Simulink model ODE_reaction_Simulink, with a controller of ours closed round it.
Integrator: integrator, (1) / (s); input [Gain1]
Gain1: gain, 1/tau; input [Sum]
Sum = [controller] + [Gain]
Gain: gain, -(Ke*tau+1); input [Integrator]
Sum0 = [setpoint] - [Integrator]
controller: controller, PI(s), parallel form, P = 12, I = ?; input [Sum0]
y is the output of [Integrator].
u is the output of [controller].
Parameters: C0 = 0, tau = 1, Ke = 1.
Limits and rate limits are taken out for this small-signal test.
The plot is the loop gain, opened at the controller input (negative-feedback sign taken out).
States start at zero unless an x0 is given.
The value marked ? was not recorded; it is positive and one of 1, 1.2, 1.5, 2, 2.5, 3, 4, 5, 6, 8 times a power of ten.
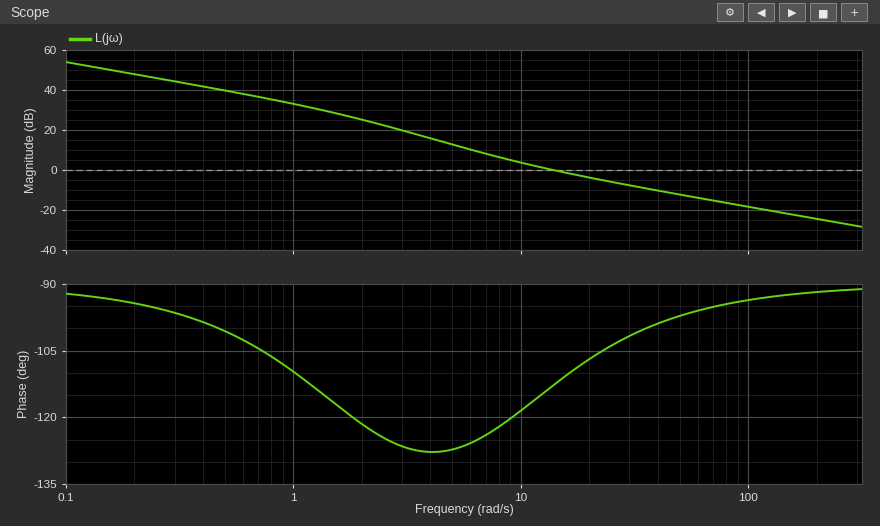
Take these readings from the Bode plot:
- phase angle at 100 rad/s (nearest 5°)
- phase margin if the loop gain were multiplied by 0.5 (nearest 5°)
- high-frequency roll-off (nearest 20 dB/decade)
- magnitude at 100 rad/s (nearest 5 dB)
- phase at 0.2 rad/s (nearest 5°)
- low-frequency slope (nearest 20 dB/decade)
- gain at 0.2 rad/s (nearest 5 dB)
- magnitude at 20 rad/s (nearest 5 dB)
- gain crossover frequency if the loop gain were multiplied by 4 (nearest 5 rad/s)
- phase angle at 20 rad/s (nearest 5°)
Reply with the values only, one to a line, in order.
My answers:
-95°
60°
-20 dB/decade
-20 dB
-95°
-20 dB/decade
50 dB
-5 dB
50 rad/s
-105°
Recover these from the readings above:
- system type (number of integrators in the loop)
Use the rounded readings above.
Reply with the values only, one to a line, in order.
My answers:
1
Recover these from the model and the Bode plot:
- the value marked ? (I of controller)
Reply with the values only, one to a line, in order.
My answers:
100
